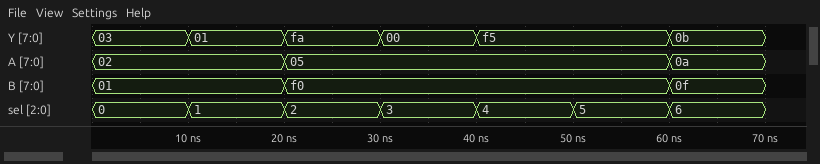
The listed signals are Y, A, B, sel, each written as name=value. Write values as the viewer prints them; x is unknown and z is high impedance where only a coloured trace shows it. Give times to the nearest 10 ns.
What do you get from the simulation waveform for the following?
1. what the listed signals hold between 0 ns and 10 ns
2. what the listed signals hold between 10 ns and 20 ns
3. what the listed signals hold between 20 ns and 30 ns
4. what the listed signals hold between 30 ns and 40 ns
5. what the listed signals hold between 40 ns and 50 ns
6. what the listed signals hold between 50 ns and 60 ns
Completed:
Y=03, A=02, B=01, sel=0
Y=01, A=02, B=01, sel=1
Y=fa, A=05, B=f0, sel=2
Y=00, A=05, B=f0, sel=3
Y=f5, A=05, B=f0, sel=4
Y=f5, A=05, B=f0, sel=5
